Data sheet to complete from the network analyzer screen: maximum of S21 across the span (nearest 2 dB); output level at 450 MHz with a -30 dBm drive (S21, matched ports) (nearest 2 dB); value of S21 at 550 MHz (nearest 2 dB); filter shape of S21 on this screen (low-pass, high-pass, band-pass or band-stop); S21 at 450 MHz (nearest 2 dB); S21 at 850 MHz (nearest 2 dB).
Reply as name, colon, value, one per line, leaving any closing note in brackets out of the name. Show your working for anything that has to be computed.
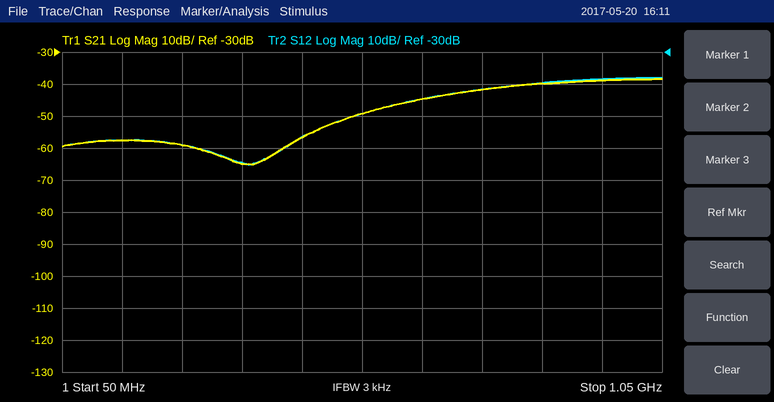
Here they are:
maximum of S21 across the span: -38 dB
output level at 450 MHz with a -30 dBm drive (S21, matched ports): -30 dBm + (-56 dB) = -86 dBm
value of S21 at 550 MHz: -50 dB
filter shape of S21 on this screen: high-pass
S21 at 450 MHz: -56 dB
S21 at 850 MHz: -40 dB
